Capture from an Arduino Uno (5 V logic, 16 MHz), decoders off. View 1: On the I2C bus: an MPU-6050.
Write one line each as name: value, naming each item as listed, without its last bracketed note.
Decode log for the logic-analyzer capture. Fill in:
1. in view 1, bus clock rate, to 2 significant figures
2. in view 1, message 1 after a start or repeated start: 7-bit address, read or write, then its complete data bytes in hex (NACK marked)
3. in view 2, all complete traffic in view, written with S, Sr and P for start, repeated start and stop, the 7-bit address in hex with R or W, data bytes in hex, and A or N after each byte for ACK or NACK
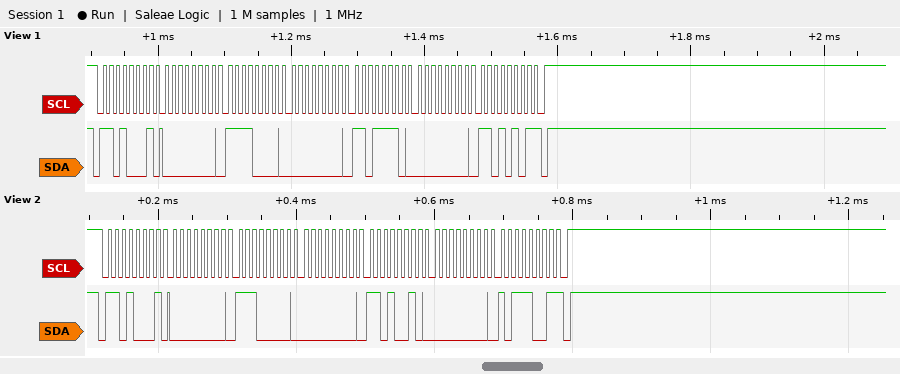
in view 1, bus clock rate, to 2 significant figures: 100 kHz
in view 1, message 1 after a start or repeated start: 7-bit address, read or write, then its complete data bytes in hex: 0x68 read: 00 F0 00 DE 00 D5 NACK
in view 2, all complete traffic in view, written with S, Sr and P for start, repeated start and stop, the 7-bit address in hex with R or W, data bytes in hex, and A or N after each byte for ACK or NACK: S 68R A 00 A E0 A 00 A D2 A 00 A B9 N P
